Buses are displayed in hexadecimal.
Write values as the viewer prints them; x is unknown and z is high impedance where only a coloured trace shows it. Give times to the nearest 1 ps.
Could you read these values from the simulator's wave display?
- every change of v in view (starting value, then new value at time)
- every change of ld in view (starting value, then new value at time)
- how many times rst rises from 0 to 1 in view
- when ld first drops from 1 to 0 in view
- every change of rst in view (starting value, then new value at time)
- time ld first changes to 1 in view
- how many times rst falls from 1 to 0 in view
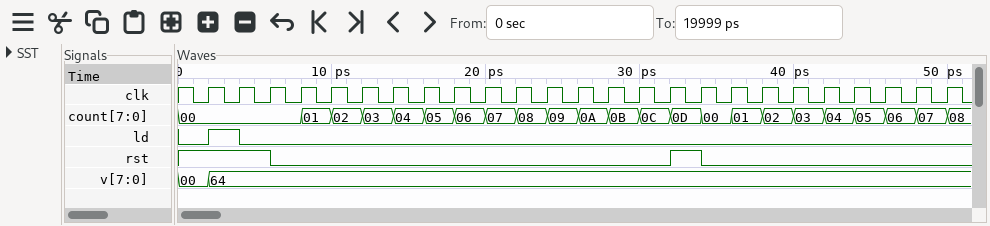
00, 64 at 2 ps
0, 1 at 2 ps, 0 at 4 ps
1
4 ps
1, 0 at 6 ps, 1 at 32 ps, 0 at 34 ps
2 ps
2
